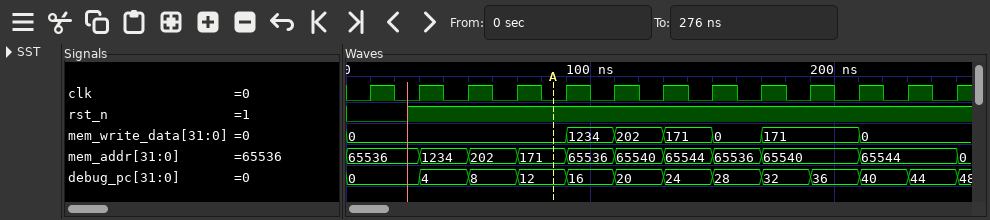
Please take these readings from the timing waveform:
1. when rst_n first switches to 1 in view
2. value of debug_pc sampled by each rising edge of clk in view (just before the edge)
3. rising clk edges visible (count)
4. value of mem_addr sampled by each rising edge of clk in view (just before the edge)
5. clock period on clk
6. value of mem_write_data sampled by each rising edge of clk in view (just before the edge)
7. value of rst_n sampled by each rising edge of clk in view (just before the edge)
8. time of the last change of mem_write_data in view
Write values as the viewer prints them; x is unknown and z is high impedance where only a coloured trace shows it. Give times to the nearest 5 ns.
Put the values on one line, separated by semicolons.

25 ns; 0, 0, 4, 8, 12, 16, 20, 24, 28, 32, 36, 40, 44; 13; 65536, 65536, 1234, 202, 171, 65536, 65540, 65544, 65536, 65540, 65540, 65544, 65544; 20 ns; 0, 0, 0, 0, 0, 1234, 202, 171, 0, 171, 171, 0, 0; 0 1 1 1 1 1 1 1 1 1 1 1 1; 210 ns
